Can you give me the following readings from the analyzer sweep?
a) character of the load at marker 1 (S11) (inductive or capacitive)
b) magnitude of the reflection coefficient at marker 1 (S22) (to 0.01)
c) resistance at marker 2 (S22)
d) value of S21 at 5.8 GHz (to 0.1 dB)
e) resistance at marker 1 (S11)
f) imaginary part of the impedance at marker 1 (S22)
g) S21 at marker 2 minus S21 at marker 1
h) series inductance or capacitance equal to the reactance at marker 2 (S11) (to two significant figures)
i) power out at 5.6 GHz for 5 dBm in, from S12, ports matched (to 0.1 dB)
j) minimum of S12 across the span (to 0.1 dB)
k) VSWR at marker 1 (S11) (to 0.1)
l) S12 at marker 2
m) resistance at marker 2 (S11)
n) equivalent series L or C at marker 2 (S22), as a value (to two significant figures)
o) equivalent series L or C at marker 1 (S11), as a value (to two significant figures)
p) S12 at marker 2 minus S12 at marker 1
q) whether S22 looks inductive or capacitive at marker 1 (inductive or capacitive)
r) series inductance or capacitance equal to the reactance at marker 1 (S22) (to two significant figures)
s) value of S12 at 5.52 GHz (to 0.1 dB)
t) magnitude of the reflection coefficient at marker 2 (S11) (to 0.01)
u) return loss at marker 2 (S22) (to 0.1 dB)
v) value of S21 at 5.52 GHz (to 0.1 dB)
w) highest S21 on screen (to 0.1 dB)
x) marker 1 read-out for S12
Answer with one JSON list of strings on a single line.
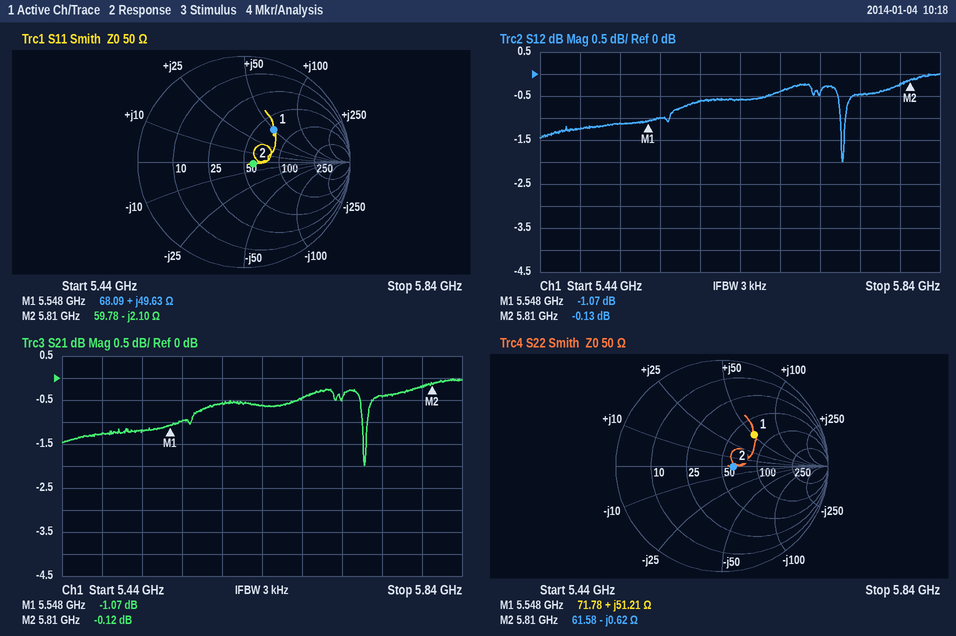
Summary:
["inductive", "0.42", "61.58 Ω", "-0.2 dB", "68.09 Ω", "+51.21 Ω", "0.95 dB", "13 pF", "4.4 dBm", "-2.0 dB", "2.4", "-0.13 dB", "59.78 Ω", "44 pF", "1.4 nH", "0.94 dB", "inductive", "1.5 nH", "-1.1 dB", "0.09", "19.7 dB", "-1.2 dB", "0.0 dB", "-1.07 dB"]
